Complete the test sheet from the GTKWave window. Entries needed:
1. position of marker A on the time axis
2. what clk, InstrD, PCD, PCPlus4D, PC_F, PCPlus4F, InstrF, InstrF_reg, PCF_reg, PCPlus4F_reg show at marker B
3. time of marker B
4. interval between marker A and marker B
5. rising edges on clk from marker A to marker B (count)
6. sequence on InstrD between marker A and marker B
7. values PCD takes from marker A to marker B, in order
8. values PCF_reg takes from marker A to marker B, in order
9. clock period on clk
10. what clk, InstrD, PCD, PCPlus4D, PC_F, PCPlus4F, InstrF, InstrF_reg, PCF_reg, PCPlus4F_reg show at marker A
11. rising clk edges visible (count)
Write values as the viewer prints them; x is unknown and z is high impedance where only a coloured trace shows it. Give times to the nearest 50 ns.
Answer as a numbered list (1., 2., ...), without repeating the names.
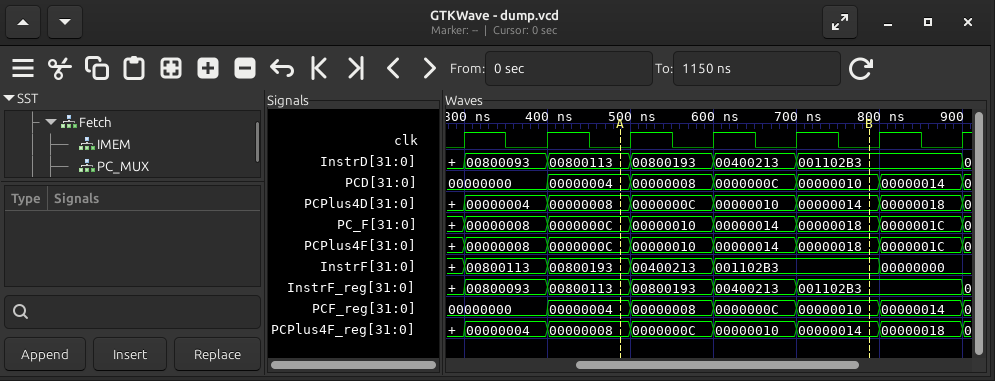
1. 500 ns
2. clk=0, InstrD=001102B3, PCD=00000010, PCPlus4D=00000014, PC_F=00000018, PCPlus4F=00000018, InstrF=001102B3, InstrF_reg=001102B3, PCF_reg=00000010, PCPlus4F_reg=00000014
3. 800 ns
4. 300 ns
5. 3
6. 00800113, 00800193, 00400213, 001102B3
7. 00000004, 00000008, 0000000C, 00000010
8. 00000004, 00000008, 0000000C, 00000010
9. 100 ns
10. clk=0, InstrD=00800113, PCD=00000004, PCPlus4D=00000008, PC_F=0000000C, PCPlus4F=0000000C, InstrF=00800193, InstrF_reg=00800113, PCF_reg=00000004, PCPlus4F_reg=00000008
11. 7
